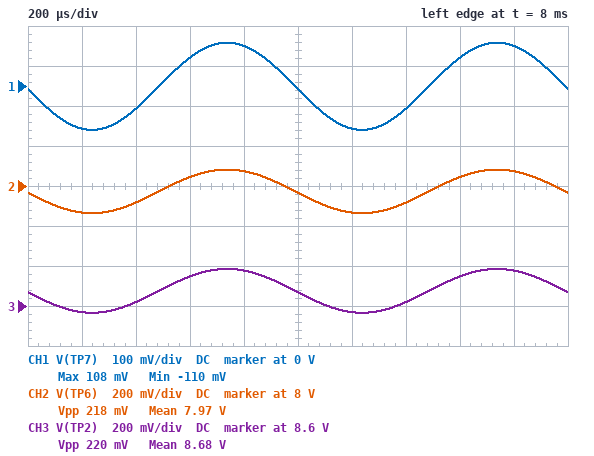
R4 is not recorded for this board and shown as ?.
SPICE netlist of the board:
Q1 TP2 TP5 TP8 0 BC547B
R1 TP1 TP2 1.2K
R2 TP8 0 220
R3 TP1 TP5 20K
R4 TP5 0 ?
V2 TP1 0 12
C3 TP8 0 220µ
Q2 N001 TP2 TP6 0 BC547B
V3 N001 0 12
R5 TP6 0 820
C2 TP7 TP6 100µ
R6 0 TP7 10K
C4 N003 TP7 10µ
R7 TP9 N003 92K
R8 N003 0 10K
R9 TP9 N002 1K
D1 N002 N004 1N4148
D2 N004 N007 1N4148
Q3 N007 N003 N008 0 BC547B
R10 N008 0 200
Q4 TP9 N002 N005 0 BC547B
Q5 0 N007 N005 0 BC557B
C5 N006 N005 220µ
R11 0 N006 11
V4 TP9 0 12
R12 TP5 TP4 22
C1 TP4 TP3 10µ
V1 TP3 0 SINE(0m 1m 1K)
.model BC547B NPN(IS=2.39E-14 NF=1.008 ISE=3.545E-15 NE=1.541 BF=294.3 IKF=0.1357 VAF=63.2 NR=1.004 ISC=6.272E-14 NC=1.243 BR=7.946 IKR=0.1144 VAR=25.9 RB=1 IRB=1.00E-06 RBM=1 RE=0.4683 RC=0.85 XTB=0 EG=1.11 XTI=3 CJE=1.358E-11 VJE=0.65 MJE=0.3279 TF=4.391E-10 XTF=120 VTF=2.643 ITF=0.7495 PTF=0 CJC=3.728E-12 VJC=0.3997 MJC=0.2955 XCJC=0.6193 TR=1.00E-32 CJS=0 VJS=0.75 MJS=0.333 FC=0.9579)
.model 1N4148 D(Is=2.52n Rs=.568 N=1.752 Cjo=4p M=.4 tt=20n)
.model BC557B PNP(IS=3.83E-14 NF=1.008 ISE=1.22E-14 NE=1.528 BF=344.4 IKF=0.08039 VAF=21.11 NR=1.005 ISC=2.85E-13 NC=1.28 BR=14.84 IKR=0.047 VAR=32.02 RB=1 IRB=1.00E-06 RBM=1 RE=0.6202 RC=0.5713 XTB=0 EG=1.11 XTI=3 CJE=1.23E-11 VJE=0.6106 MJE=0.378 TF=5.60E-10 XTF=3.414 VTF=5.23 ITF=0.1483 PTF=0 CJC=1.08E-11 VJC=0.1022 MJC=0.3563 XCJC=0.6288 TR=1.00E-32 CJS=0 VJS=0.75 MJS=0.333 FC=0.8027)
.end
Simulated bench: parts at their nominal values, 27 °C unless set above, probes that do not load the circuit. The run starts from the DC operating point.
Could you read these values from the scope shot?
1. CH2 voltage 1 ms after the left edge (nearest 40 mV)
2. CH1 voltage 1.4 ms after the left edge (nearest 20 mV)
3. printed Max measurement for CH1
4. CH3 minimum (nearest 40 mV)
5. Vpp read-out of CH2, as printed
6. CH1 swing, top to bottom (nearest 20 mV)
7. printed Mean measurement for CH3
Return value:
7.96 V
-60 mV
108 mV
8.56 V
218 mV
220 mV
8.68 V
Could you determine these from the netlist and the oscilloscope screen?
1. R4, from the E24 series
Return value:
2.4 kΩ
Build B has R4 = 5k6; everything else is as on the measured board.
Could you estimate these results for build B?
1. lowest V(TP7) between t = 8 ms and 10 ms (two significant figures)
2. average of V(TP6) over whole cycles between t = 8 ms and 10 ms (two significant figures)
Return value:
-240 mV
1.6 V
